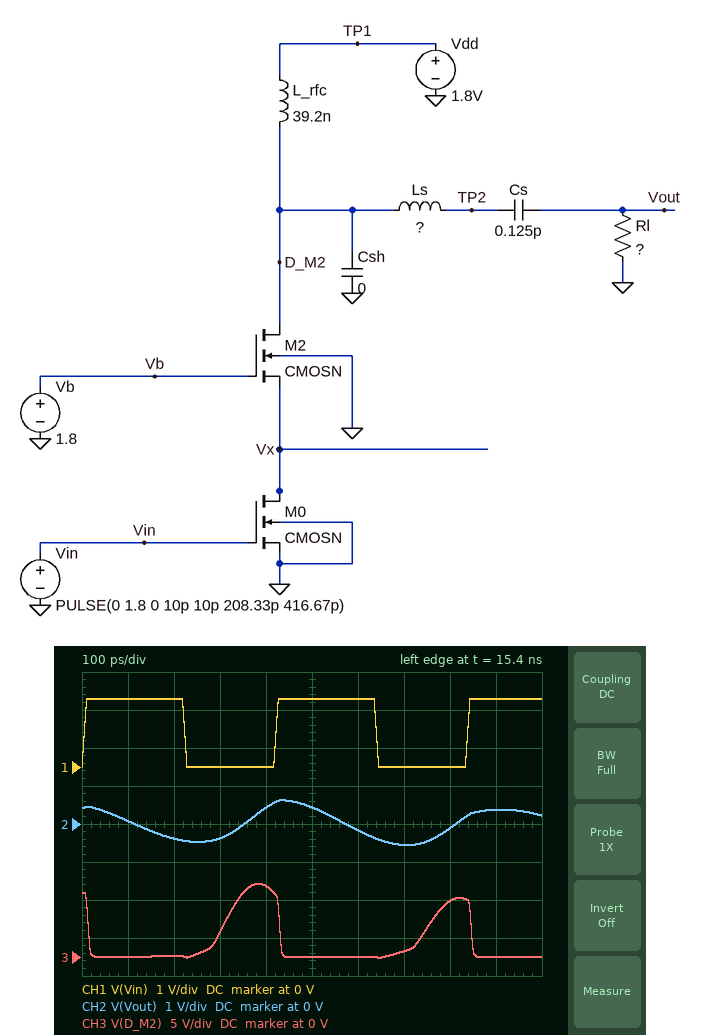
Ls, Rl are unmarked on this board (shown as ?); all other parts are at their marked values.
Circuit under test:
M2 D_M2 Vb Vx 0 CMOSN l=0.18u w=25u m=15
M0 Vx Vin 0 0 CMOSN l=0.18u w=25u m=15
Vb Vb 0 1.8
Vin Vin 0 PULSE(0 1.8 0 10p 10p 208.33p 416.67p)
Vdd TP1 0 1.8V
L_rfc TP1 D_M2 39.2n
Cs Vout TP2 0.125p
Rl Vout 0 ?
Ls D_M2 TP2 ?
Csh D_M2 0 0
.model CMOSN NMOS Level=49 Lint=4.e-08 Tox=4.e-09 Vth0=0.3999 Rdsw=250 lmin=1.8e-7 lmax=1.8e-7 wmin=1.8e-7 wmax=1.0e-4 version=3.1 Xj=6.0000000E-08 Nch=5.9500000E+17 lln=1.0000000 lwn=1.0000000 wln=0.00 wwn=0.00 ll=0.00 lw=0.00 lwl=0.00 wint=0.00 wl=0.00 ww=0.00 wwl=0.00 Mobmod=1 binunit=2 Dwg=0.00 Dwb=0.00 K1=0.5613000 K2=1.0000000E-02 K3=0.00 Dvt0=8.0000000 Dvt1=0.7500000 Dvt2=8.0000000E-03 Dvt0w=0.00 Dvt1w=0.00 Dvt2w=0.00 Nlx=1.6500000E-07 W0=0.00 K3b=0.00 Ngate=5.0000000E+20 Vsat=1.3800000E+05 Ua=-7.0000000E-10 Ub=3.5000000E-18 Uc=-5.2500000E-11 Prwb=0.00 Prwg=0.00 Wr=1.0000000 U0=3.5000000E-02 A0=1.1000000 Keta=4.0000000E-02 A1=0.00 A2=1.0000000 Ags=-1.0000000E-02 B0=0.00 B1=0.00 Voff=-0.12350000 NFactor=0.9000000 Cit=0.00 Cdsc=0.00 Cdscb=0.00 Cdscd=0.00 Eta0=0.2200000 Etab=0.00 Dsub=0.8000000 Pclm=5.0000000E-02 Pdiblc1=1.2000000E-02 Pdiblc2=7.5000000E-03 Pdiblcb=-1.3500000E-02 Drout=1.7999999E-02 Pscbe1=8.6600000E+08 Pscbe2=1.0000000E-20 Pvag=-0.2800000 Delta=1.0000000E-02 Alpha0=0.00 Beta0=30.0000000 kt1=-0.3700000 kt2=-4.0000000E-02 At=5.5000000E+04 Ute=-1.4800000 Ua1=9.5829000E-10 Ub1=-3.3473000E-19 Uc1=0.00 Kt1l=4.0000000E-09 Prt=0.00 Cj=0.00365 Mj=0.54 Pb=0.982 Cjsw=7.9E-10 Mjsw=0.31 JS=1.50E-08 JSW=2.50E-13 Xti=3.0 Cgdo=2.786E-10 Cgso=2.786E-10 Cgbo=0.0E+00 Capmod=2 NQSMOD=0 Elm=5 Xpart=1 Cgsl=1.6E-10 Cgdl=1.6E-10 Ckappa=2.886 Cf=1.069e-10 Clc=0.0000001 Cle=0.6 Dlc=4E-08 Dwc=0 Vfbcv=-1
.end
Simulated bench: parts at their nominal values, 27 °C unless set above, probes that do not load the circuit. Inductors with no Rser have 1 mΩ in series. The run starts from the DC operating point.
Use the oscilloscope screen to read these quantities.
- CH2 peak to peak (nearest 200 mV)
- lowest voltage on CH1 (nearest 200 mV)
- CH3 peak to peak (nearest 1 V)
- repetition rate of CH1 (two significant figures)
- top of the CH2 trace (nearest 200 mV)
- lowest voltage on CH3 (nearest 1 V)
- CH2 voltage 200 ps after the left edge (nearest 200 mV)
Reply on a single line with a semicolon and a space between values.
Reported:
1.2 V; 0 V; 10 V; 2.4 GHz; 600 mV; 0 V; -400 mV
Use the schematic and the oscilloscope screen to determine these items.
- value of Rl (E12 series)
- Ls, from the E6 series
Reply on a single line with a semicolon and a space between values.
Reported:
47 Ω; 68 nH
